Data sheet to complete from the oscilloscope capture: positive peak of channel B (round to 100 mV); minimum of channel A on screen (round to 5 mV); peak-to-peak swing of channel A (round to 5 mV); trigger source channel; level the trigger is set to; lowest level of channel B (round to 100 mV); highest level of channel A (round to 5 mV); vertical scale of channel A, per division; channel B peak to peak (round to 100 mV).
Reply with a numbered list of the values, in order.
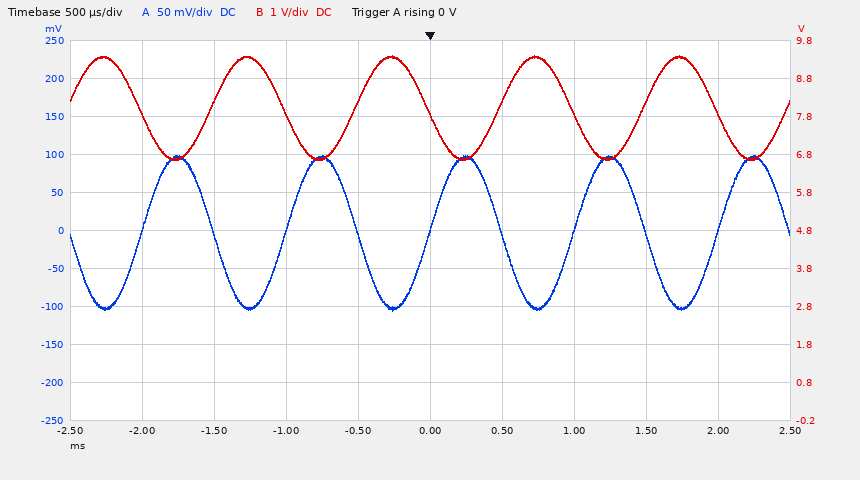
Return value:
1. 9.4 V
2. -105 mV
3. 205 mV
4. channel A
5. 0 V
6. 6.7 V
7. 100 mV
8. 50 mV
9. 2.7 V
